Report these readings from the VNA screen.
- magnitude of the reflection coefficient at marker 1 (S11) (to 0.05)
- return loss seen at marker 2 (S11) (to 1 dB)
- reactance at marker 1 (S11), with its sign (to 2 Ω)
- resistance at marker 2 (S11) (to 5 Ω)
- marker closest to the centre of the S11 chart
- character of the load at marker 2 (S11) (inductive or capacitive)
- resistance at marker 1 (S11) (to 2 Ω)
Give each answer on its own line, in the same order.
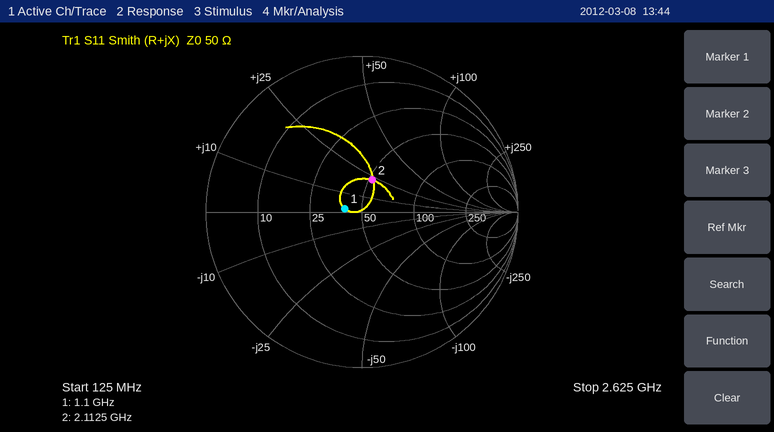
0.10
13 dB
+2 Ω
50 Ω
marker 1
inductive
40 Ω
